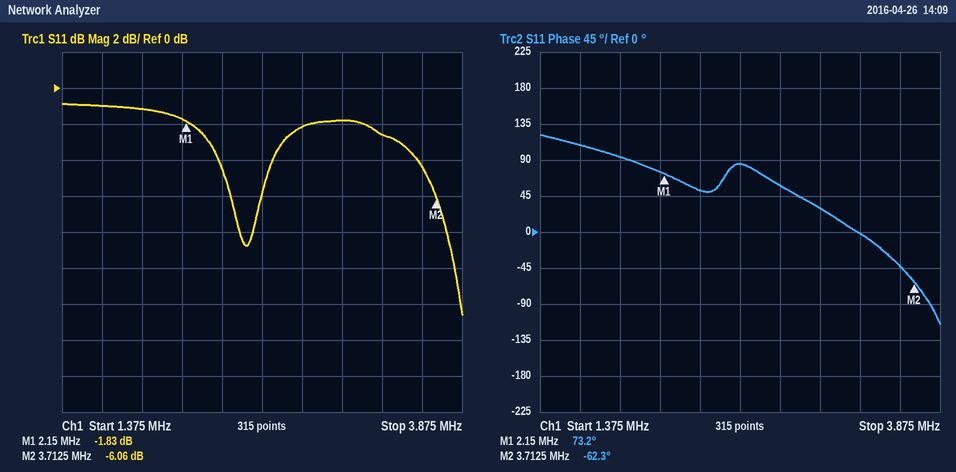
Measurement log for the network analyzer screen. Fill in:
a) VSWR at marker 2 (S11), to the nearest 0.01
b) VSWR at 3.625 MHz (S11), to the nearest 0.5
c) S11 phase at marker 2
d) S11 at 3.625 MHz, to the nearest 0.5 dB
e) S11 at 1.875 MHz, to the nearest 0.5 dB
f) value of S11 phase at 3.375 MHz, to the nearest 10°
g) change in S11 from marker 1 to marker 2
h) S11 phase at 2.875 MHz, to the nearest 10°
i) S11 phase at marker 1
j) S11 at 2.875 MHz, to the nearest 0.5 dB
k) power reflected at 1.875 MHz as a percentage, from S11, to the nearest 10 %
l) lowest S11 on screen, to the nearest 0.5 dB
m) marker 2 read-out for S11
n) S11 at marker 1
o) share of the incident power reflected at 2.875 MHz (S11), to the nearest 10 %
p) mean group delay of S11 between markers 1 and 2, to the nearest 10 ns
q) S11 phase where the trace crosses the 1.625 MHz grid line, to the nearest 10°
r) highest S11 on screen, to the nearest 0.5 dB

2.98
4.0
-62.3°
-4.5 dB
-1.0 dB
0°
-4.23 dB
60°
73.2°
-2.0 dB
80 %
-12.5 dB
-6.06 dB
-1.83 dB
60 %
240 ns
110°
-1.0 dB
